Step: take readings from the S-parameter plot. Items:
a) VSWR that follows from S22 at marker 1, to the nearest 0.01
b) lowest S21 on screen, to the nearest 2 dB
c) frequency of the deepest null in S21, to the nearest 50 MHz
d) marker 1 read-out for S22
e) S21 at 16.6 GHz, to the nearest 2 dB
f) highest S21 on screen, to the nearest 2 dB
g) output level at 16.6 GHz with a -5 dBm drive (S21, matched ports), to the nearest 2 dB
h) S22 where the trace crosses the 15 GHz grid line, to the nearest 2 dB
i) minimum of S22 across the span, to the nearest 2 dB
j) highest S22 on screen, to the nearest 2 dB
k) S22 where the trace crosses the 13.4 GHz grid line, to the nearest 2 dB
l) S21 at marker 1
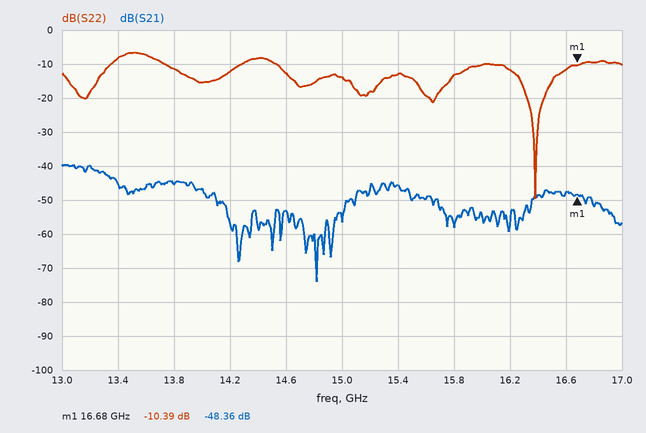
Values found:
1.87
-74 dB
14.80 GHz
-10.39 dB
-48 dB
-40 dB
-52 dBm
-14 dB
-50 dB
-6 dB
-8 dB
-48.36 dB
